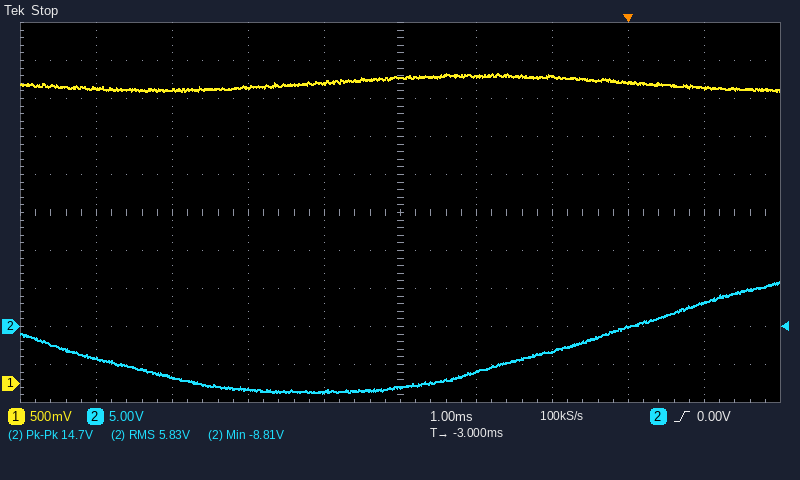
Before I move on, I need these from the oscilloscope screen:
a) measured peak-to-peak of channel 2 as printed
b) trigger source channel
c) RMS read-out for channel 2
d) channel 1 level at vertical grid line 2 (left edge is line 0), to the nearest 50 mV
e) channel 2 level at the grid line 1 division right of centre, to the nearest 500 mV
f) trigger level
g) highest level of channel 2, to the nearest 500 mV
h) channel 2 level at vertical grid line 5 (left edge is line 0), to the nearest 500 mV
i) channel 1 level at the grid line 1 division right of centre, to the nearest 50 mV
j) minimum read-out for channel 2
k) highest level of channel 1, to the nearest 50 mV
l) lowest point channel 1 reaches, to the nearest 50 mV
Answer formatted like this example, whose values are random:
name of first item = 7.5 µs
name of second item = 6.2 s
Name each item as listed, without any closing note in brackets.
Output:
measured peak-to-peak of channel 2 as printed = 14.7 V
trigger source channel = channel 2
RMS read-out for channel 2 = 5.83 V
channel 1 level at vertical grid line 2 (left edge is line 0), to the nearest 50 mV = 3.85 V
channel 2 level at the grid line 1 division right of centre, to the nearest 500 mV = -6.0 V
trigger level = 0.00 V
highest level of channel 2, to the nearest 500 mV = 6.0 V
channel 2 level at vertical grid line 5 (left edge is line 0), to the nearest 500 mV = -8.0 V
channel 1 level at the grid line 1 division right of centre, to the nearest 50 mV = 4.05 V
minimum read-out for channel 2 = -8.81 V
highest level of channel 1, to the nearest 50 mV = 4.10 V
lowest point channel 1 reaches, to the nearest 50 mV = 3.85 V
